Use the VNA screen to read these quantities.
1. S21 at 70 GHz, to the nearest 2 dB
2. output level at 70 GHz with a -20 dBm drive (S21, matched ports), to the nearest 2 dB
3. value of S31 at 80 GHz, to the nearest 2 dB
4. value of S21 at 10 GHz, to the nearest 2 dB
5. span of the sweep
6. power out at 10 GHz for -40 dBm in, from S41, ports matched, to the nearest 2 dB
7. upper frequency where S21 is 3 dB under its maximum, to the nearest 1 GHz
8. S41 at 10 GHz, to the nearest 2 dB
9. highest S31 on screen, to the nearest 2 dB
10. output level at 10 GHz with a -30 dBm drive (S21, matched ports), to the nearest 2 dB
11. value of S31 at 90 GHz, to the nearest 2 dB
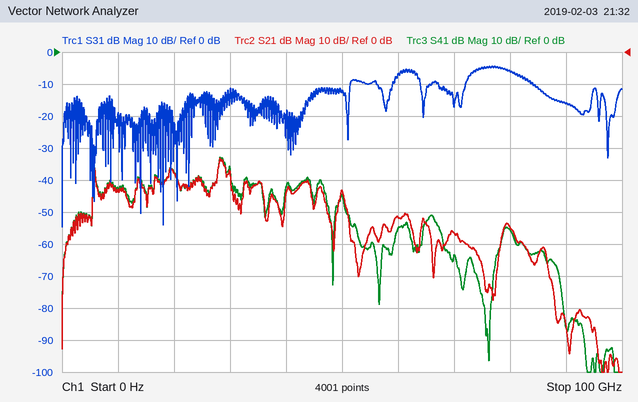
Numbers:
-56 dB
-76 dBm
-6 dB
-44 dB
100 GHz
-82 dBm
29 GHz
-42 dB
-4 dB
-74 dBm
-16 dB
